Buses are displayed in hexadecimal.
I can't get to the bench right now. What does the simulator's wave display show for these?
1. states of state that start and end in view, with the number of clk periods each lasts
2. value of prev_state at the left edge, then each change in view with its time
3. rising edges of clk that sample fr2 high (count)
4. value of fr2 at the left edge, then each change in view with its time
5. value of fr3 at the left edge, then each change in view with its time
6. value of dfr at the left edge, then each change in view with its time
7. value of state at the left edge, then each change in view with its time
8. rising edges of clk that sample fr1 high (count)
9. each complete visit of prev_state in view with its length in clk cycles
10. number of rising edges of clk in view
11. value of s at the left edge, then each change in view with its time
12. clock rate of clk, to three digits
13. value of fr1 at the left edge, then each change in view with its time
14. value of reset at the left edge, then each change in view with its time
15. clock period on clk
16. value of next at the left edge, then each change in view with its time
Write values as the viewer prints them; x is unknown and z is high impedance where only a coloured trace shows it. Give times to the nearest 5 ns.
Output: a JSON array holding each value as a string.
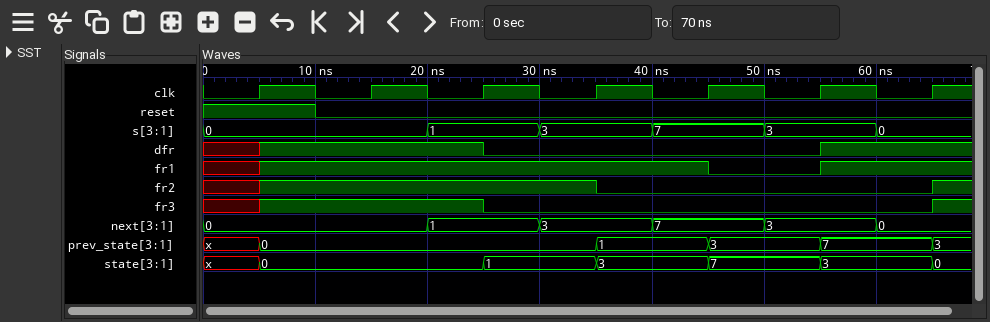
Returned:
["0: 2, 1: 1, 3: 1, 7: 1, 3: 1", "x, 0 at 5 ns, 1 at 35 ns, 3 at 45 ns, 7 at 55 ns, 3 at 65 ns", "3", "x, 1 at 5 ns, 0 at 35 ns, 1 at 65 ns", "x, 1 at 5 ns, 0 at 25 ns, 1 at 65 ns", "x, 1 at 5 ns, 0 at 25 ns, 1 at 55 ns", "x, 0 at 5 ns, 1 at 25 ns, 3 at 35 ns, 7 at 45 ns, 3 at 55 ns, 0 at 65 ns", "5", "0: 3, 1: 1, 3: 1, 7: 1", "7", "0, 1 at 20 ns, 3 at 30 ns, 7 at 40 ns, 3 at 50 ns, 0 at 60 ns", "100 MHz", "x, 1 at 5 ns, 0 at 45 ns, 1 at 55 ns", "1, 0 at 10 ns", "10 ns", "0, 1 at 20 ns, 3 at 30 ns, 7 at 40 ns, 3 at 50 ns, 0 at 60 ns"]
